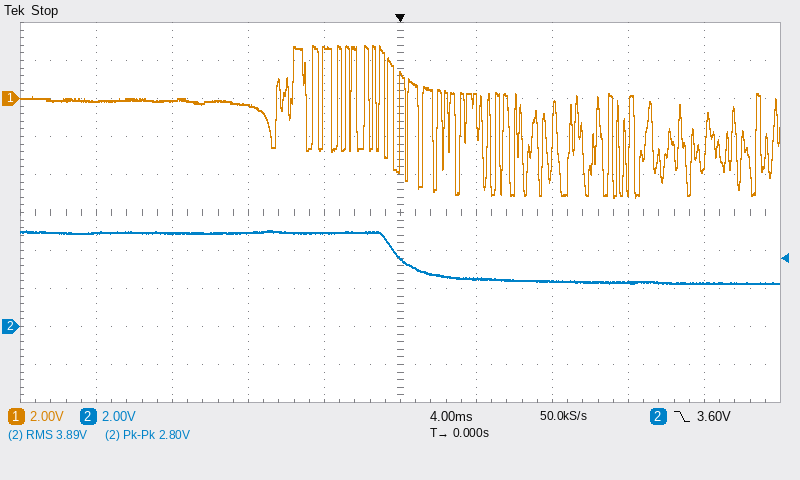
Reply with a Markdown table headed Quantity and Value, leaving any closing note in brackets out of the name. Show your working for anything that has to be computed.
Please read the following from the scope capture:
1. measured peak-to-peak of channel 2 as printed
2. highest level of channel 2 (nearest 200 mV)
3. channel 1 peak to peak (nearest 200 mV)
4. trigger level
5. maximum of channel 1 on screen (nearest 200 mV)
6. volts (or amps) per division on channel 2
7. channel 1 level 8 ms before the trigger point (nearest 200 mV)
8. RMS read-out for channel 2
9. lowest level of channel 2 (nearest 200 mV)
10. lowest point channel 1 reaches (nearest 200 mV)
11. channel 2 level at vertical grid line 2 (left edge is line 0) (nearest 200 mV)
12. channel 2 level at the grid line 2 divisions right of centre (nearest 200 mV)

| Quantity | Value |
|---|---|
| measured peak-to-peak of channel 2 as printed | 2.80 V |
| highest level of channel 2 | 5.0 V |
| channel 1 peak to peak | 2.8 V − (-5.2 V) = 8.0 V |
| trigger level | 3.60 V |
| maximum of channel 1 on screen | 2.8 V |
| volts (or amps) per division on channel 2 | 2 V |
| channel 1 level 8 ms before the trigger point | -400 mV |
| RMS read-out for channel 2 | 3.89 V |
| lowest level of channel 2 | 2.2 V |
| lowest point channel 1 reaches | -5.2 V |
| channel 2 level at vertical grid line 2 (left edge is line 0) | 5.0 V |
| channel 2 level at the grid line 2 divisions right of centre | 2.4 V |
